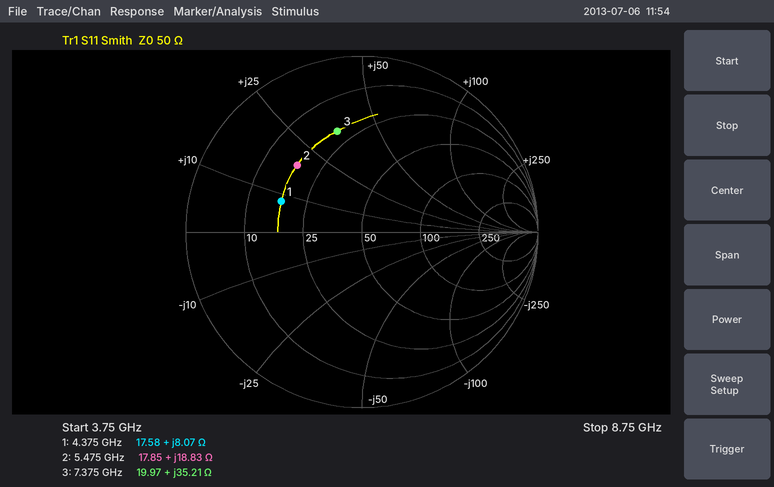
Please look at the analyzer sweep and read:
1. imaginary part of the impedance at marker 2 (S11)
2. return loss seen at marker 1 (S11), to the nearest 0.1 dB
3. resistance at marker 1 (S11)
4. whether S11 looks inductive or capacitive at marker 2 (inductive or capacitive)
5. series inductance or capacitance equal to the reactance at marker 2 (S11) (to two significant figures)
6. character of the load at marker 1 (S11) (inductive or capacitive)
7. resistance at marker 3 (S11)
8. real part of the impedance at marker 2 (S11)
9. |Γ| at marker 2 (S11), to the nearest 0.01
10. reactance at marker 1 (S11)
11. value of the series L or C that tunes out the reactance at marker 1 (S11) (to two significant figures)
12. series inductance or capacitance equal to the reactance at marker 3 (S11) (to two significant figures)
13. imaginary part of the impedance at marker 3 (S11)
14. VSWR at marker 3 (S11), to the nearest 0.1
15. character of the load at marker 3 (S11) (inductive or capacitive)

+18.83 Ω
6.2 dB
17.58 Ω
inductive
550 pH
inductive
19.97 Ω
17.85 Ω
0.53
+8.07 Ω
4.5 pF
760 pH
+35.21 Ω
3.9
inductive
